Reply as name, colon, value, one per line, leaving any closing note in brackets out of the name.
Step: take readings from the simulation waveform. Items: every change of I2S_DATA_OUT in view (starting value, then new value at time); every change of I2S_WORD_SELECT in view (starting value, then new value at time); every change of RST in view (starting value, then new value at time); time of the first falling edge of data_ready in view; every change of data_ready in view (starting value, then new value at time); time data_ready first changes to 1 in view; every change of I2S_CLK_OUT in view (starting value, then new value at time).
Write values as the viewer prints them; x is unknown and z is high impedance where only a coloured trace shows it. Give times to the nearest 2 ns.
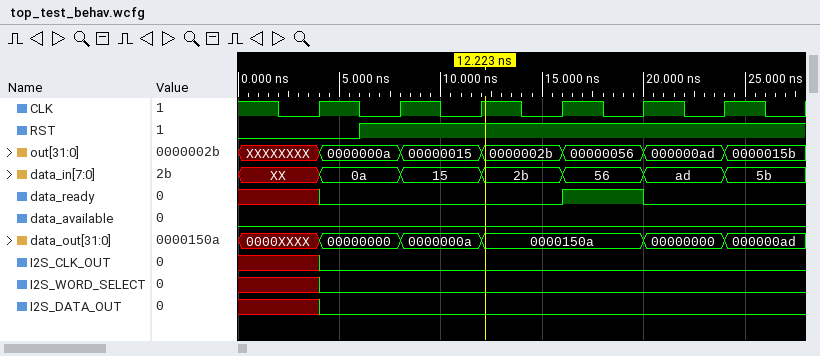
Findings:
every change of I2S_DATA_OUT in view: x, 0 at 4 ns
every change of I2S_WORD_SELECT in view: x, 0 at 4 ns
every change of RST in view: 0, 1 at 6 ns
time of the first falling edge of data_ready in view: 20 ns
every change of data_ready in view: x, 0 at 4 ns, 1 at 16 ns, 0 at 20 ns
time data_ready first changes to 1 in view: 16 ns
every change of I2S_CLK_OUT in view: x, 0 at 4 ns
